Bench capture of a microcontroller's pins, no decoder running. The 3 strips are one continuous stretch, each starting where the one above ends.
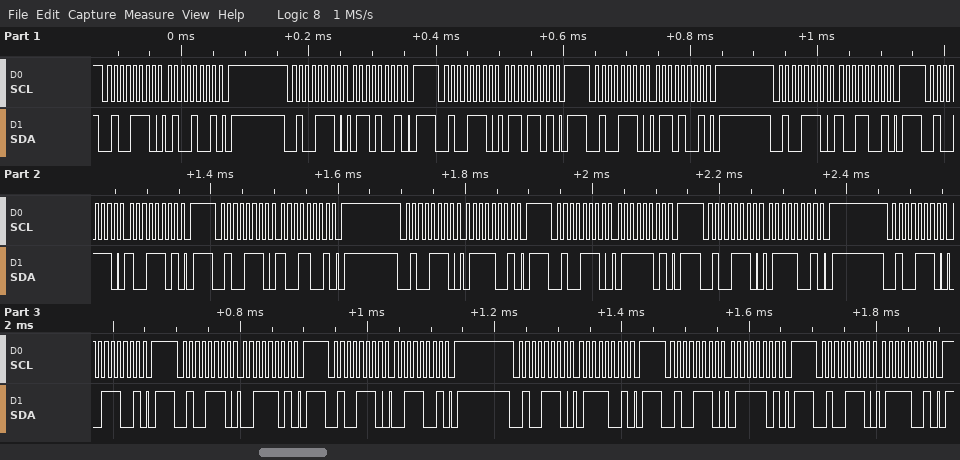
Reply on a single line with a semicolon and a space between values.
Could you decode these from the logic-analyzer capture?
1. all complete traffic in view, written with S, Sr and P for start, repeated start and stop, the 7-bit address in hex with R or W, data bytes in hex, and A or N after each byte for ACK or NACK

S 27W A 49 A P S 27W A 69 A P S 27W A 6D A P S 27W A 69 A P S 27W A 99 A P S 27W A 9D A P S 27W A 99 A P S 27W A 79 A P S 27W A 7D A P S 27W A 79 A P S 27W A 39 A P S 27W A 3D A P S 27W A 39 A P S 27W A 79 A P S 27W A 7D A P S 27W A 79 A P
